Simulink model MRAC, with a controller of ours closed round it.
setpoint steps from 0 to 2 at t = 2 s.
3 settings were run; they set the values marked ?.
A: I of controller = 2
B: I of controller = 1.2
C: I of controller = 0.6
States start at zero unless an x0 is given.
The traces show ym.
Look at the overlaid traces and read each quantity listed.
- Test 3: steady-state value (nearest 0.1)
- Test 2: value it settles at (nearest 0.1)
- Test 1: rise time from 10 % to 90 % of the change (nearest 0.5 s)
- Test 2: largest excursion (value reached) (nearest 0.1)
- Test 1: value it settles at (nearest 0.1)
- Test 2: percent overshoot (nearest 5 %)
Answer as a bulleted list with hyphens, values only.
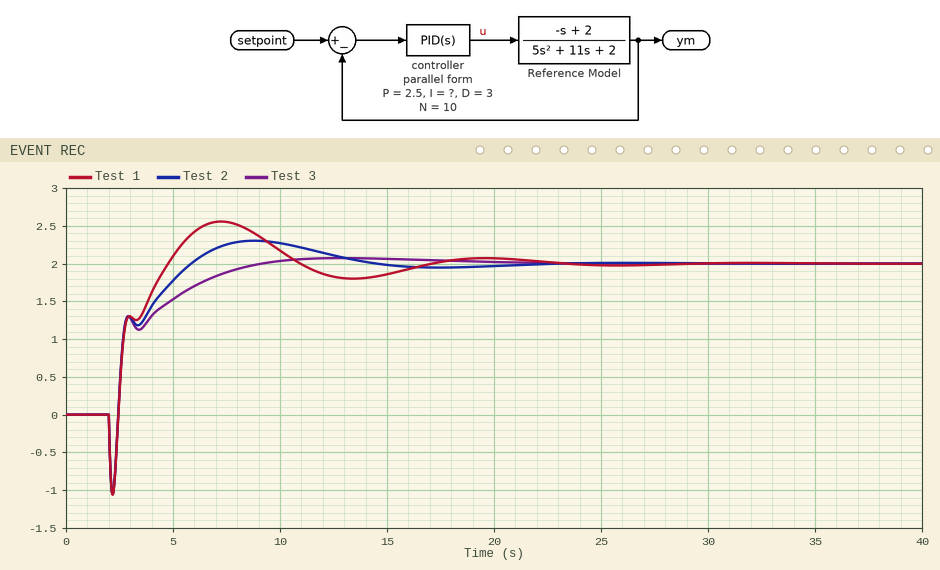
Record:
- 2.0
- 2.0
- 2.0 s
- 2.3
- 2.0
- 15 %
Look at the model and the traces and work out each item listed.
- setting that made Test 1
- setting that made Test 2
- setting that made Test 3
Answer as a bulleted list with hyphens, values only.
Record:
- A
- B
- C
